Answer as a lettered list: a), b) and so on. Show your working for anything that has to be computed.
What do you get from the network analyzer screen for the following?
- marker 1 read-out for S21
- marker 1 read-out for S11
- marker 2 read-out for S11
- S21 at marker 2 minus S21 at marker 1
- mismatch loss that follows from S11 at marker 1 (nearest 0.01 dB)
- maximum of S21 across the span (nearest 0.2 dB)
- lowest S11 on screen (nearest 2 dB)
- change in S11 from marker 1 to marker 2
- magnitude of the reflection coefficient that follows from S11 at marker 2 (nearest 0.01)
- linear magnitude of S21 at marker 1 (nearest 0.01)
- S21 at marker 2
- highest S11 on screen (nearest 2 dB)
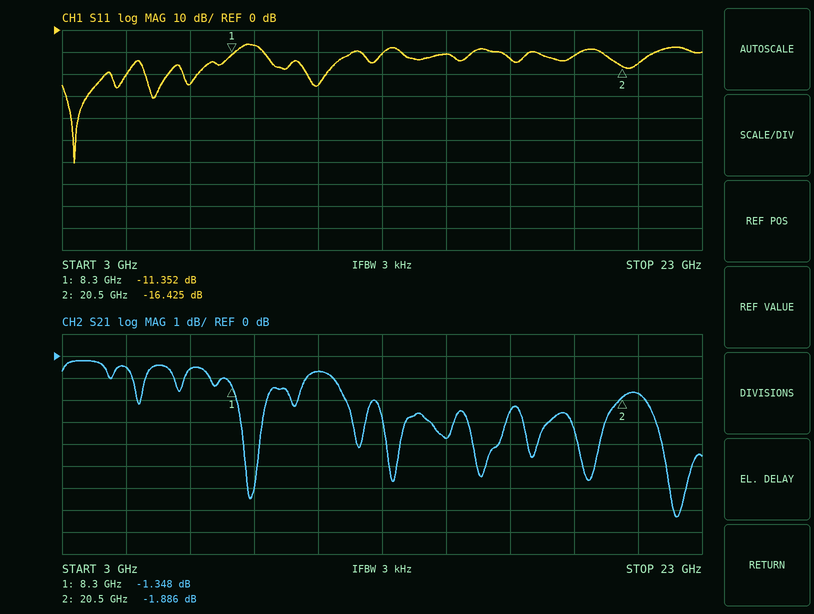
a) -1.348 dB
b) -11.352 dB
c) -16.425 dB
d) -1.886 − (-1.348) = -0.538 dB
e) −10 log10(1 − 10^(-11.352/10)) ≈ 0.33 dB
f) -0.2 dB
g) -60 dB
h) -16.425 − (-11.352) = -5.073 dB
i) 10^(-16.425/20) ≈ 0.15
j) 10^(-1.348/20) ≈ 0.86
k) -1.886 dB
l) -6 dB
